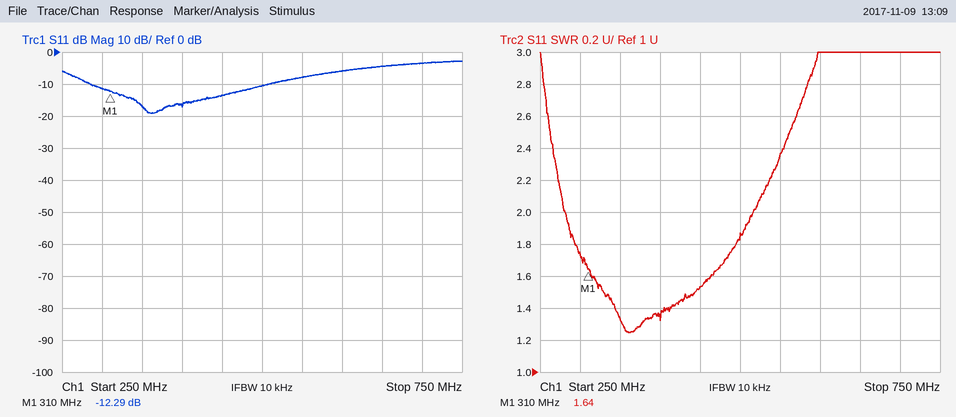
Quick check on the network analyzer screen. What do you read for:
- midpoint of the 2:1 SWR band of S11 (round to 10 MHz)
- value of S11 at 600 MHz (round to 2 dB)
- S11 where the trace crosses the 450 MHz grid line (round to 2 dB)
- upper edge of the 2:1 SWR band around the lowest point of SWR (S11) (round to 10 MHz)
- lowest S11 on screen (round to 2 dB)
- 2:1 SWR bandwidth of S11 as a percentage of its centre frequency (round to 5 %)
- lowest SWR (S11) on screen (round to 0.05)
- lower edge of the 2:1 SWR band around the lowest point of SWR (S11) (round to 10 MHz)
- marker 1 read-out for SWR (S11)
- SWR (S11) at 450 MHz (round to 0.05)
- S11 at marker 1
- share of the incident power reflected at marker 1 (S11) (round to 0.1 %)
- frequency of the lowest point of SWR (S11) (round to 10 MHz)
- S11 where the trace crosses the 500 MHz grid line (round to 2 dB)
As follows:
400 MHz
-6 dB
-14 dB
520 MHz
-20 dB
60 %
1.25
280 MHz
1.64
1.55
-12.29 dB
5.9 %
360 MHz
-10 dB
